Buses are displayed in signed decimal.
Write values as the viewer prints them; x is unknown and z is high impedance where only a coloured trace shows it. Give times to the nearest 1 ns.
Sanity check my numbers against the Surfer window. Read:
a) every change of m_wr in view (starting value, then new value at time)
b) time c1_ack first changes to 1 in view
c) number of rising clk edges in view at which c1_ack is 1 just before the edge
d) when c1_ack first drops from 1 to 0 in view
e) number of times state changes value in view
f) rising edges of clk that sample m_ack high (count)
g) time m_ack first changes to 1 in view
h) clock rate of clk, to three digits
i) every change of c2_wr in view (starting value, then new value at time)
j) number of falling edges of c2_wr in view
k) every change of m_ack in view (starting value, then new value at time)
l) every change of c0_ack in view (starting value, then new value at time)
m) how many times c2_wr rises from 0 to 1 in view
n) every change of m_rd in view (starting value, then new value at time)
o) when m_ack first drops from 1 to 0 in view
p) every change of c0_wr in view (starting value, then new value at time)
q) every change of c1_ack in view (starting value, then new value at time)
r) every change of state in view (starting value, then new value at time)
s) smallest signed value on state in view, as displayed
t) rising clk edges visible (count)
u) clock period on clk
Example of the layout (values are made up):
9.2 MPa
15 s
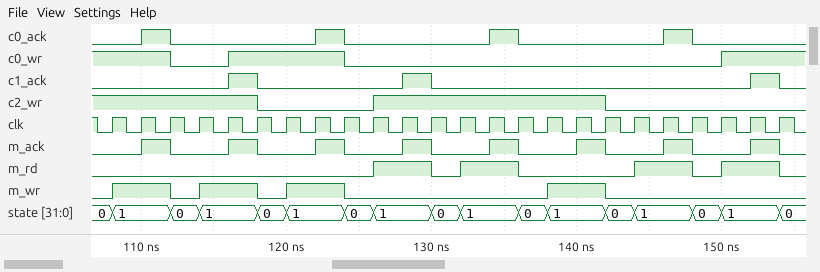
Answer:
0, 1 at 108 ns, 0 at 112 ns, 1 at 114 ns, 0 at 118 ns, 1 at 120 ns, 0 at 124 ns, 1 at 138 ns, 0 at 142 ns
116 ns
3
118 ns
16
8
110 ns
500 MHz
1, 0 at 118 ns, 1 at 126 ns, 0 at 142 ns
2
0, 1 at 110 ns, 0 at 112 ns, 1 at 116 ns, 0 at 118 ns, 1 at 122 ns, 0 at 124 ns, 1 at 128 ns, 0 at 130 ns, 1 at 134 ns, 0 at 136 ns, 1 at 140 ns, 0 at 142 ns, 1 at 146 ns, 0 at 148 ns, 1 at 152 ns, 0 at 154 ns
0, 1 at 110 ns, 0 at 112 ns, 1 at 122 ns, 0 at 124 ns, 1 at 134 ns, 0 at 136 ns, 1 at 146 ns, 0 at 148 ns
1
0, 1 at 126 ns, 0 at 130 ns, 1 at 132 ns, 0 at 136 ns, 1 at 144 ns, 0 at 148 ns, 1 at 150 ns, 0 at 154 ns
112 ns
1, 0 at 112 ns, 1 at 116 ns, 0 at 124 ns, 1 at 150 ns
0, 1 at 116 ns, 0 at 118 ns, 1 at 128 ns, 0 at 130 ns, 1 at 152 ns, 0 at 154 ns
0, 1 at 108 ns, 0 at 112 ns, 1 at 114 ns, 0 at 118 ns, 1 at 120 ns, 0 at 124 ns, 1 at 126 ns, 0 at 130 ns, 1 at 132 ns, 0 at 136 ns, 1 at 138 ns, 0 at 142 ns, 1 at 144 ns, 0 at 148 ns, 1 at 150 ns, 0 at 154 ns
0
24
2 ns
